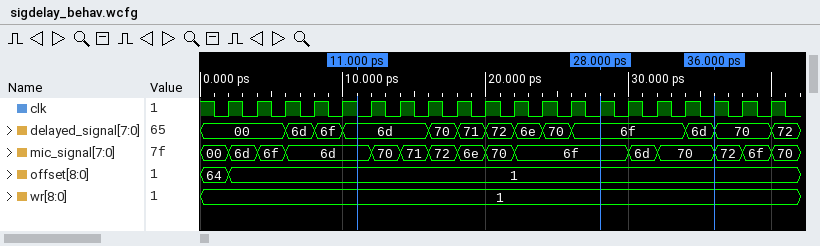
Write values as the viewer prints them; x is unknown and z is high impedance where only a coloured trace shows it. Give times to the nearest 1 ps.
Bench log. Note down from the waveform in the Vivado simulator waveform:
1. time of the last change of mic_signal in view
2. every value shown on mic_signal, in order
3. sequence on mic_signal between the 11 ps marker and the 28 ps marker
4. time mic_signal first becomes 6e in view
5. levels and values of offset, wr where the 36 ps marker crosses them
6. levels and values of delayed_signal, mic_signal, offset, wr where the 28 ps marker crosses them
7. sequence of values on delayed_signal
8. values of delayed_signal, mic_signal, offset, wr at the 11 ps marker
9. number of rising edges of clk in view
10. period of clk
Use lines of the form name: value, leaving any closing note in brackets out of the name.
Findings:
time of the last change of mic_signal in view: 40 ps
every value shown on mic_signal, in order: 00, 6d, 6f, 6d, 70, 71, 72, 6e, 70, 6f, 6d, 70, 72, 6f, 70
sequence on mic_signal between the 11 ps marker and the 28 ps marker: 6d, 70, 71, 72, 6e, 70, 6f
time mic_signal first becomes 6e in view: 18 ps
levels and values of offset, wr where the 36 ps marker crosses them: offset=1, wr=1
levels and values of delayed_signal, mic_signal, offset, wr where the 28 ps marker crosses them: delayed_signal=6f, mic_signal=6f, offset=1, wr=1
sequence of values on delayed_signal: 00, 6d, 6f, 6d, 70, 71, 72, 6e, 70, 6f, 6d, 70, 72
values of delayed_signal, mic_signal, offset, wr at the 11 ps marker: delayed_signal=6d, mic_signal=6d, offset=1, wr=1
number of rising edges of clk in view: 20
period of clk: 2 ps
